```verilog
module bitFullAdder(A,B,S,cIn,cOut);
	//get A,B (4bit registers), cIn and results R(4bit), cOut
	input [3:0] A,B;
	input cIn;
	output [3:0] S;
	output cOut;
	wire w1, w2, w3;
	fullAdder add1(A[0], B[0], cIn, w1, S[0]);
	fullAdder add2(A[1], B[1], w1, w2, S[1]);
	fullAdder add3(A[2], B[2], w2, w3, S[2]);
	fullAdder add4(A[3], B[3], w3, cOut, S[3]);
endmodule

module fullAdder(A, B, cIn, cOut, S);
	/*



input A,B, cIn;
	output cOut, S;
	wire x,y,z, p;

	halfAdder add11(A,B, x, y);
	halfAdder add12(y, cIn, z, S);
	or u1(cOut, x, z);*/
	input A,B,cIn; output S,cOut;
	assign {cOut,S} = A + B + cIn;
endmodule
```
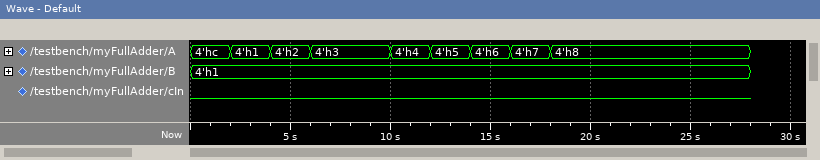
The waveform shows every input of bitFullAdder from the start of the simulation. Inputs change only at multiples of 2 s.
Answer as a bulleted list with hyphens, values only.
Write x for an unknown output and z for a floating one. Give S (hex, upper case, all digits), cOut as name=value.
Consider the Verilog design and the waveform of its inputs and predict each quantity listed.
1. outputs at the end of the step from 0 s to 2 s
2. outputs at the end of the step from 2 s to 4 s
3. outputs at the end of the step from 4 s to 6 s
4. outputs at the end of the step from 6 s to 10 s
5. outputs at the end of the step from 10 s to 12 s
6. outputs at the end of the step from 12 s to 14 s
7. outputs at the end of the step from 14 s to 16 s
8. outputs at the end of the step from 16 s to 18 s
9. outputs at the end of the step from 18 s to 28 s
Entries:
- S=D, cOut=0
- S=2, cOut=0
- S=3, cOut=0
- S=4, cOut=0
- S=5, cOut=0
- S=6, cOut=0
- S=7, cOut=0
- S=8, cOut=0
- S=9, cOut=0
